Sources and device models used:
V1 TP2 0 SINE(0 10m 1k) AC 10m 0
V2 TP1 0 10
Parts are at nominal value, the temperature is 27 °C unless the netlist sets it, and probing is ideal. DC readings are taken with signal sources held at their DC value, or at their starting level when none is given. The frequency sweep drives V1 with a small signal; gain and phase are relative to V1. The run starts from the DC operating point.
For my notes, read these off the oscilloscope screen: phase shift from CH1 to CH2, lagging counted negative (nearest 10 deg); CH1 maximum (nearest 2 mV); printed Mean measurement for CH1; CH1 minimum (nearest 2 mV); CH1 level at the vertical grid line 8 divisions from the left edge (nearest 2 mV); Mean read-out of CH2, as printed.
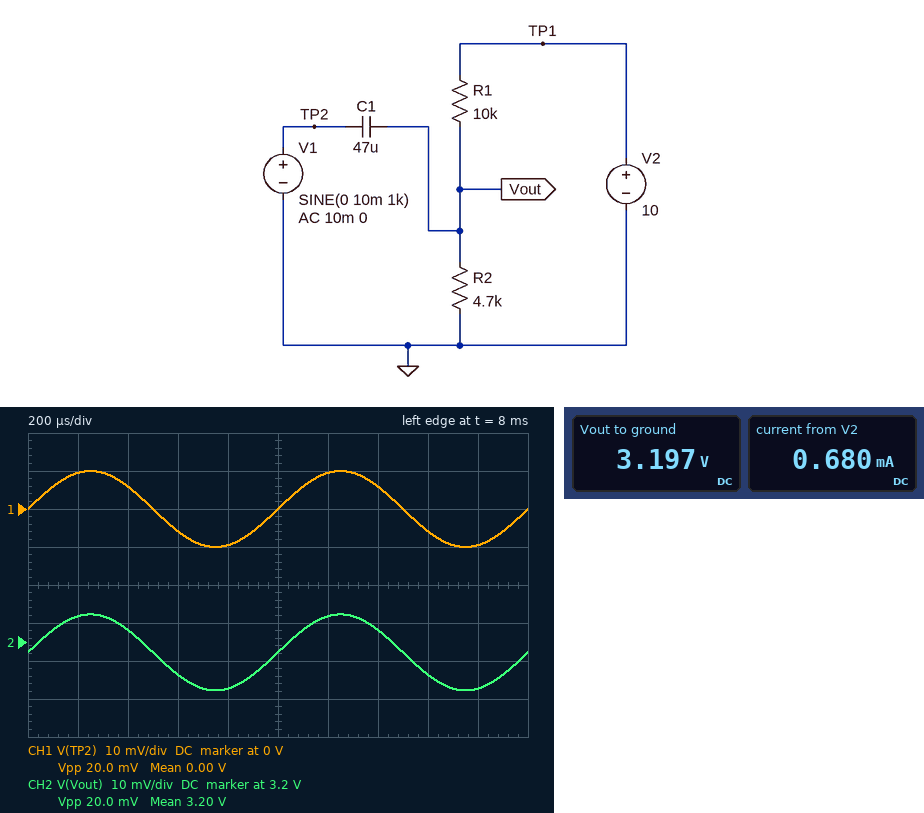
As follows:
0 deg
10 mV
0.00 V
-10 mV
-6 mV
3.20 V
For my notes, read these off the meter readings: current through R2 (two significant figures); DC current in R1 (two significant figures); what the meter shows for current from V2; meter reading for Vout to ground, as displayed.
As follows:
680 µA
680 µA
0.680 mA
3.197 V
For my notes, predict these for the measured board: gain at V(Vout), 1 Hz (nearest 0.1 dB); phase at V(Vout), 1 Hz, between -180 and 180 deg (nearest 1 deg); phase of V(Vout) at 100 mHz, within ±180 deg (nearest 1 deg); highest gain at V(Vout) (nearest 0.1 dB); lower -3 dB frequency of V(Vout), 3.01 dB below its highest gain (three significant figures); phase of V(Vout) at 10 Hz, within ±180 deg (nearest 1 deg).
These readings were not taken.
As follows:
-3.3 dB
47 deg
85 deg
0 dB
1.06 Hz
6 deg
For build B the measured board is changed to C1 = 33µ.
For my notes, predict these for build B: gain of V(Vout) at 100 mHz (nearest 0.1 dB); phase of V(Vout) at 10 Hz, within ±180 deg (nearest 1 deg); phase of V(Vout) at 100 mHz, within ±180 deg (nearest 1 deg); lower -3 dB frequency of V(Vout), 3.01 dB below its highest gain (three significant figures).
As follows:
-23.6 dB
9 deg
86 deg
1.51 Hz
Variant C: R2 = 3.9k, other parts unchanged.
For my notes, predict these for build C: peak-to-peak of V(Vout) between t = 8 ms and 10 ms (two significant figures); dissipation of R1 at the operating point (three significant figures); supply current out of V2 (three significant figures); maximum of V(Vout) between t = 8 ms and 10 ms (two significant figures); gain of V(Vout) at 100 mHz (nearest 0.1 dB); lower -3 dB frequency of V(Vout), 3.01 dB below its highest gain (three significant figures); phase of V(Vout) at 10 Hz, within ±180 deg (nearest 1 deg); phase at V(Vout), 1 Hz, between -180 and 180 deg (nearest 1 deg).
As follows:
20 mV
5.18 mW
719 µA
2.8 V
-21.7 dB
1.21 Hz
7 deg
50 deg
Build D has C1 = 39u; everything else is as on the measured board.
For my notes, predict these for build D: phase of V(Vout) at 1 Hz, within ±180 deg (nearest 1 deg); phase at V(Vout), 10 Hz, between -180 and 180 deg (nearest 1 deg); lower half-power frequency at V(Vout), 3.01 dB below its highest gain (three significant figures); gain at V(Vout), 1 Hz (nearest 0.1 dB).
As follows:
52 deg
7 deg
1.28 Hz
-4.2 dB
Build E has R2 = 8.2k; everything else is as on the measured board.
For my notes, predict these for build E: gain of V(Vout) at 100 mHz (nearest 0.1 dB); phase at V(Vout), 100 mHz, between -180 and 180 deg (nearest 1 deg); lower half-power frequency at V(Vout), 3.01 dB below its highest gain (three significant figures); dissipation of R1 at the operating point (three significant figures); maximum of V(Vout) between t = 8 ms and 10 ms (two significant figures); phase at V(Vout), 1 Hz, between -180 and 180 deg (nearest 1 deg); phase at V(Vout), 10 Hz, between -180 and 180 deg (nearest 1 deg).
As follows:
-17.6 dB
82 deg
752 mHz
3.02 mW
4.5 V
37 deg
4 deg
